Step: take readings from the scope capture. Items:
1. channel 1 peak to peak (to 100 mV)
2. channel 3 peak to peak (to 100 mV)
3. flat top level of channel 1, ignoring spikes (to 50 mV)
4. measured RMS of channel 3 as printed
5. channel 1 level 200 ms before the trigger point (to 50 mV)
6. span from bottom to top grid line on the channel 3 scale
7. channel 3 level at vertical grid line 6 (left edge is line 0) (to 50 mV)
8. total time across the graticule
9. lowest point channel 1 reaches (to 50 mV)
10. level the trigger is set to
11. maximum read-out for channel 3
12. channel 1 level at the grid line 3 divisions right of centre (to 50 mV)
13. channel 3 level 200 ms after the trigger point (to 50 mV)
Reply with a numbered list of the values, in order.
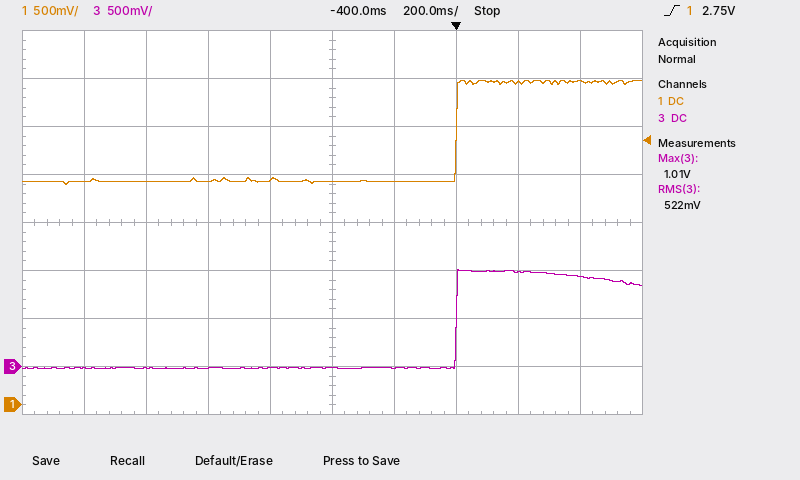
1. 1.10 V
2. 1.00 V
3. 3.35 V
4. 522 mV
5. 2.35 V
6. 4 V
7. 0 mV
8. 2 s
9. 2.30 V
10. 2.75 V
11. 1.01 V
12. 3.35 V
13. 1.00 V
